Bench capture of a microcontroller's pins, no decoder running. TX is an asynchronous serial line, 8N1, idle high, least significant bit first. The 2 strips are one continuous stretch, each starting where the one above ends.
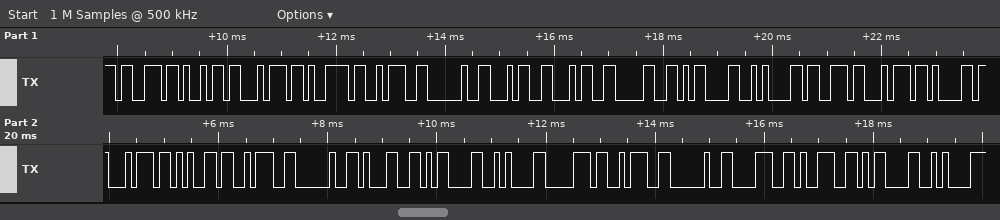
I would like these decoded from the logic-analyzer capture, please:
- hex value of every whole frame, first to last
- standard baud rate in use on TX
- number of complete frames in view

0x73 0x69 0x74 0x79 0x3A 0x20 0x34 0x34 0x30 0x0D 0x0A 0x73 0x74 0x61 0x74 0x65 0x3A 0x20 0x31 0x0D 0x0A 0x70 0x3A 0x20 0x38 0x39 0x0D 0x0A
9600 baud
28
